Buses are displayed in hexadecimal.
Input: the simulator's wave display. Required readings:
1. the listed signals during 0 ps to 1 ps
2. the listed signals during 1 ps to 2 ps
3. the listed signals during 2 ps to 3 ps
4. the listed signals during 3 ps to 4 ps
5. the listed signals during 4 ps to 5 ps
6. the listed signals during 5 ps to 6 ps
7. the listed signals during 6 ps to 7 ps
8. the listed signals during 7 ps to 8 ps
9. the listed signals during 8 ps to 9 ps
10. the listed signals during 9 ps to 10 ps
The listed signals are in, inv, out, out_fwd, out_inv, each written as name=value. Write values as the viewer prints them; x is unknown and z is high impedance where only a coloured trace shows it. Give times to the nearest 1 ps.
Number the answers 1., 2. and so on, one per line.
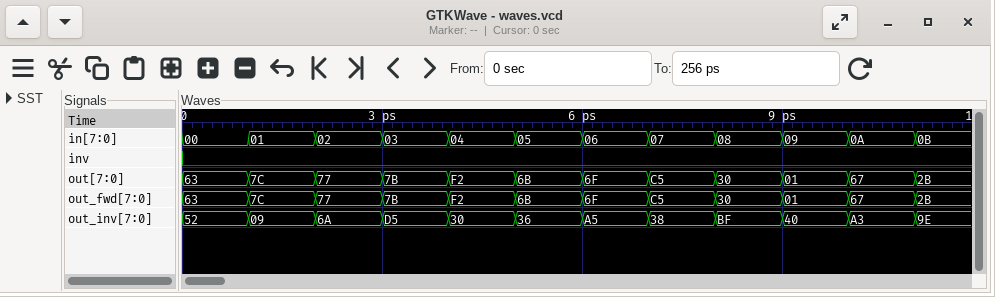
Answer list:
1. in=00, inv=0, out=63, out_fwd=63, out_inv=52
2. in=01, inv=0, out=7C, out_fwd=7C, out_inv=09
3. in=02, inv=0, out=77, out_fwd=77, out_inv=6A
4. in=03, inv=0, out=7B, out_fwd=7B, out_inv=D5
5. in=04, inv=0, out=F2, out_fwd=F2, out_inv=30
6. in=05, inv=0, out=6B, out_fwd=6B, out_inv=36
7. in=06, inv=0, out=6F, out_fwd=6F, out_inv=A5
8. in=07, inv=0, out=C5, out_fwd=C5, out_inv=38
9. in=08, inv=0, out=30, out_fwd=30, out_inv=BF
10. in=09, inv=0, out=01, out_fwd=01, out_inv=40
